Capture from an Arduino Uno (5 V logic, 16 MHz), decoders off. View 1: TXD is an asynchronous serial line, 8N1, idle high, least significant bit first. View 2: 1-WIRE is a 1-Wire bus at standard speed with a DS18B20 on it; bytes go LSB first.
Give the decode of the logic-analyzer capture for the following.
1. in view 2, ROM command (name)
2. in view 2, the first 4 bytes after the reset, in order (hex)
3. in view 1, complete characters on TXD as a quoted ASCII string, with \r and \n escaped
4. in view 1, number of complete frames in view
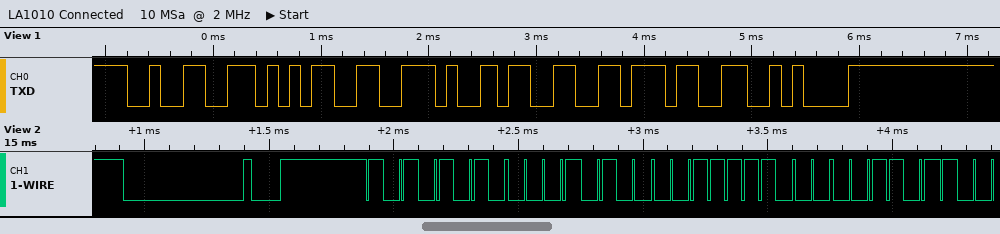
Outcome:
Match ROM
55 28 7C B0
"25.37\n"
6
